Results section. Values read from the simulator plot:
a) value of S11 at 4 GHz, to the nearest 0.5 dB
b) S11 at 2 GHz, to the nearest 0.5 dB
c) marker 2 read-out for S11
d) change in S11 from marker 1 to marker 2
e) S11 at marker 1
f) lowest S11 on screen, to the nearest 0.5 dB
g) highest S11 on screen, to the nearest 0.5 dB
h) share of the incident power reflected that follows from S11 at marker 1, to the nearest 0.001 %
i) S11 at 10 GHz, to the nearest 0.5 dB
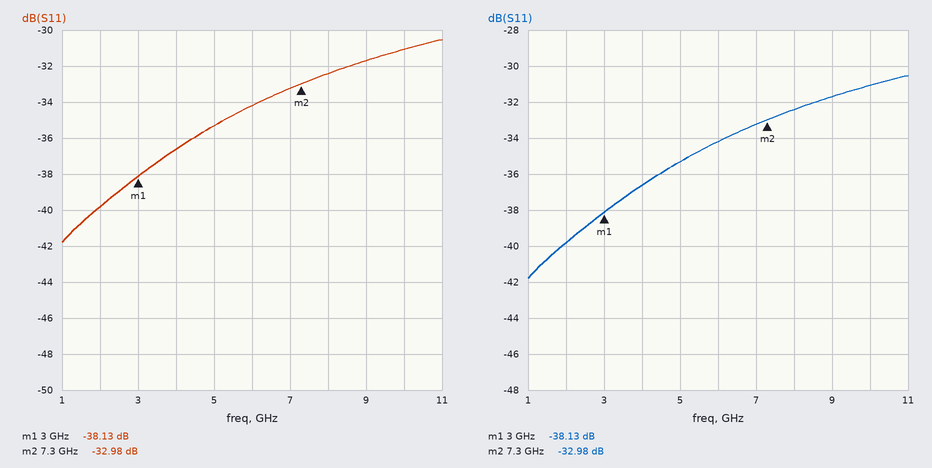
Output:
-36.5 dB
-40.0 dB
-32.98 dB
5.15 dB
-38.13 dB
-42.0 dB
-30.5 dB
0.015 %
-31.0 dB
